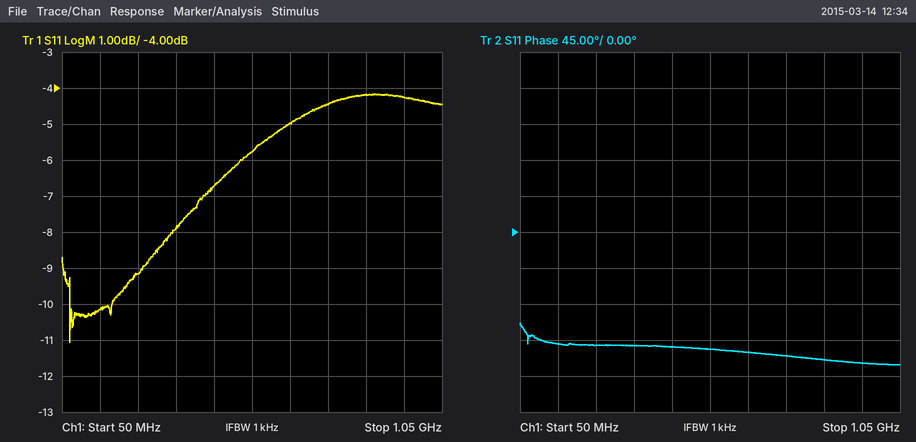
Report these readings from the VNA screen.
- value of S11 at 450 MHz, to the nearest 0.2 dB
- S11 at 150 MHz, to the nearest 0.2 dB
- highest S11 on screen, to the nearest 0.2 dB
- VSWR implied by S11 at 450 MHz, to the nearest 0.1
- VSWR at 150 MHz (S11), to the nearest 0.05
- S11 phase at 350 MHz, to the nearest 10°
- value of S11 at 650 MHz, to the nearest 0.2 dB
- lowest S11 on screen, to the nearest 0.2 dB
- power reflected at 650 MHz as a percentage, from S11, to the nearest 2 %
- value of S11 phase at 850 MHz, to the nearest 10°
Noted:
-6.8 dB
-10.2 dB
-4.2 dB
2.7
1.90
-140°
-5.0 dB
-11.0 dB
32 %
-160°
